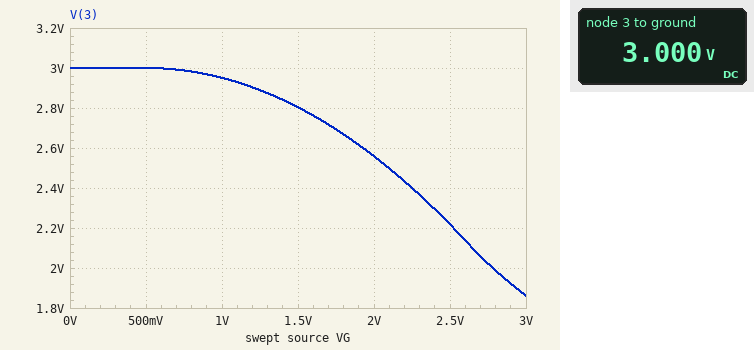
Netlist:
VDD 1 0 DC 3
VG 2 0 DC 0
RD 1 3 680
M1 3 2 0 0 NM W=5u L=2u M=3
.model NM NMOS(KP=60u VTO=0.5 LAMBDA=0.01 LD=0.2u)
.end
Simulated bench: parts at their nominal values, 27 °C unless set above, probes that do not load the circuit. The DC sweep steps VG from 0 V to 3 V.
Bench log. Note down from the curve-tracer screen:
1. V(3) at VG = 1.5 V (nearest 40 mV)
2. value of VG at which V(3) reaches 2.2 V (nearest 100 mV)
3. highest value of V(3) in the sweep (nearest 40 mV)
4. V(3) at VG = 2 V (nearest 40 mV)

2.80 V
2.5 V
3.00 V
2.56 V
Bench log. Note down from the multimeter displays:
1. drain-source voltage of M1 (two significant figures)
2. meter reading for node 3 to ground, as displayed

3.0 V
3.000 V
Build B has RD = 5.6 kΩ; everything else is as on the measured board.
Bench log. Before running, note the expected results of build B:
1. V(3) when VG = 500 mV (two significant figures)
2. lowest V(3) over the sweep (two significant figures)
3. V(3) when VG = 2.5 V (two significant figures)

3.0 V
360 mV
450 mV
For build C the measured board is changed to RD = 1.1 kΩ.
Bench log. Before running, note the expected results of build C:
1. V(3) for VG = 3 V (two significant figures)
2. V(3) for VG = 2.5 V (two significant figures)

1.4 V
1.8 V
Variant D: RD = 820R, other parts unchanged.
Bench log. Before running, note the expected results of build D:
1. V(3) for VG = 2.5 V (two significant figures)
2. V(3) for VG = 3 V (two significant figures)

2.1 V
1.7 V
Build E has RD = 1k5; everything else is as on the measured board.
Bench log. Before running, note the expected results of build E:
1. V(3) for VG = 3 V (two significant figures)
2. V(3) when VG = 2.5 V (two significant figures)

1.1 V
1.4 V
